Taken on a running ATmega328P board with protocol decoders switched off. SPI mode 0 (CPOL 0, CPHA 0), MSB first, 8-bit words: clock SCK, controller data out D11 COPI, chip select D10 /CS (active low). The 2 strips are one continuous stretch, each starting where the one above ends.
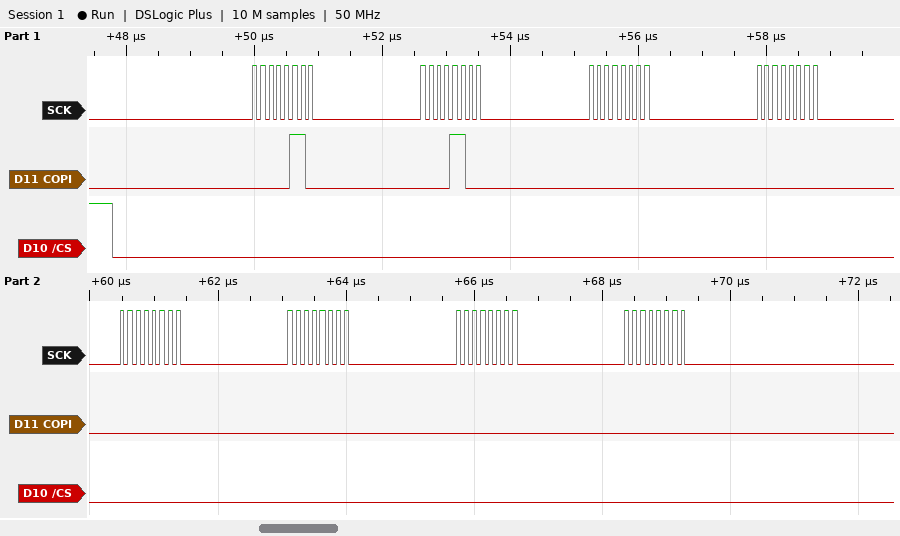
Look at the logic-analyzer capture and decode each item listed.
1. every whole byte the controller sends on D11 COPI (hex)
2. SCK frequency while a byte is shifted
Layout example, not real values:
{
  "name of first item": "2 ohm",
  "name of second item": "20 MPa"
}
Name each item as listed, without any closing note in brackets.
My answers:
{
  "every whole byte the controller sends on D11 COPI": "06 0C 00 00 00 00 00 00",
  "SCK frequency while a byte is shifted": "8 MHz"
}
